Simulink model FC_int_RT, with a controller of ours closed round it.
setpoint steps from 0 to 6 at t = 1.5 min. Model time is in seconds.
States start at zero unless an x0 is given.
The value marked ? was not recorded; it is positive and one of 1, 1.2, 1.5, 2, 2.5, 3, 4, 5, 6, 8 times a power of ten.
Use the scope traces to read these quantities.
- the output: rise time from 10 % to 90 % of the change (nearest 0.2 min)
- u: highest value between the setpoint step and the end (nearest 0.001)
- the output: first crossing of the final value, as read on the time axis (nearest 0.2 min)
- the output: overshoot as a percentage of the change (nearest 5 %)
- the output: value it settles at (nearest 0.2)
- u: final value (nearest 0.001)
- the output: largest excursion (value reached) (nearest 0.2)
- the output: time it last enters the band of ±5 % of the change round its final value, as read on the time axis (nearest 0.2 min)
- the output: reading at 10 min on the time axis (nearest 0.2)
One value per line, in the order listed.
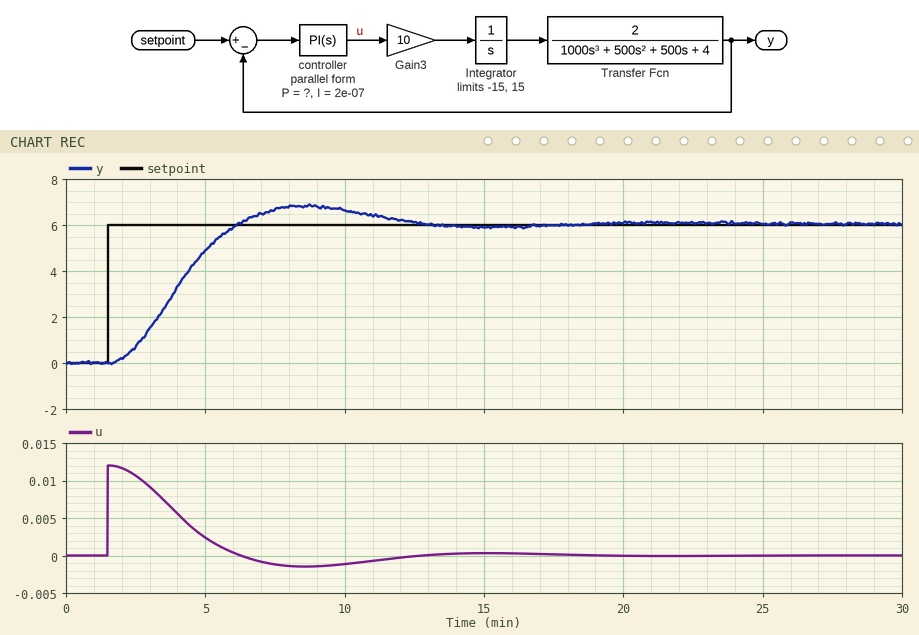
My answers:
3.0 min
0.012
6.2 min
15 %
6.0
0.000
6.8
11.4 min
6.6
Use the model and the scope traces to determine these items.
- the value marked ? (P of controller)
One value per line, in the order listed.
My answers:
0.002
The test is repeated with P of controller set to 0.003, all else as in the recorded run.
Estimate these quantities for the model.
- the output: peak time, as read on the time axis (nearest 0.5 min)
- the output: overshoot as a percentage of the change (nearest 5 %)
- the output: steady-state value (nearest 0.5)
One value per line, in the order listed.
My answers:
7.5 min
10 %
6.0
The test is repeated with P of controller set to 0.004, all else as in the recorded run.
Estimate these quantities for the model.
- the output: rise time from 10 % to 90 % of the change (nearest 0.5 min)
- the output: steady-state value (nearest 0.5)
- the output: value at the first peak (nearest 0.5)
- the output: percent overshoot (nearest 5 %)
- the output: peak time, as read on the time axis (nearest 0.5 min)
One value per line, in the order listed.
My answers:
2.5 min
6.0
6.5
10 %
7.0 min
